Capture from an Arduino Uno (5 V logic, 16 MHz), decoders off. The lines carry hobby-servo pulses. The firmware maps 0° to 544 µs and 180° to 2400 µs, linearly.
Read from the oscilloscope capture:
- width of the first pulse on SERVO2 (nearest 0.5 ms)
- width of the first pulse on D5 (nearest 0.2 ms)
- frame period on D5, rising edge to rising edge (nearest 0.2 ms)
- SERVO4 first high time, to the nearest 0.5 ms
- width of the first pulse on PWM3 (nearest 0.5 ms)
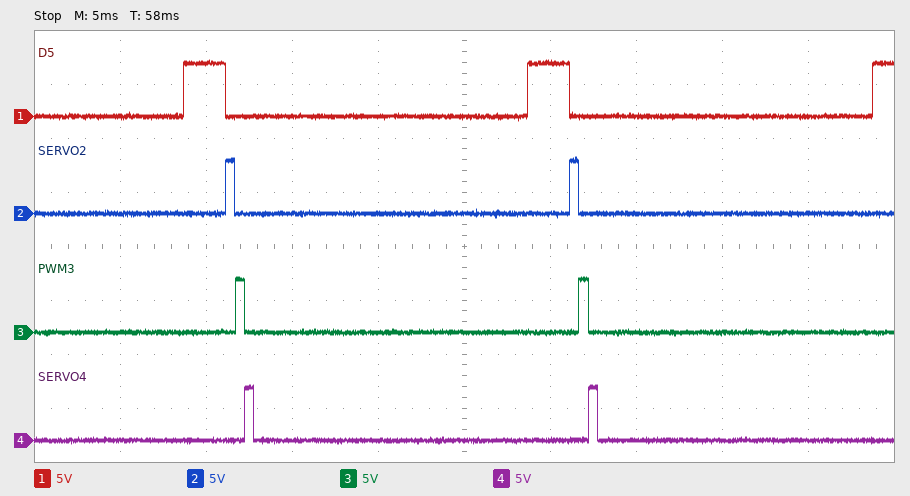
0.5 ms
2.4 ms
20.0 ms
0.5 ms
0.5 ms
